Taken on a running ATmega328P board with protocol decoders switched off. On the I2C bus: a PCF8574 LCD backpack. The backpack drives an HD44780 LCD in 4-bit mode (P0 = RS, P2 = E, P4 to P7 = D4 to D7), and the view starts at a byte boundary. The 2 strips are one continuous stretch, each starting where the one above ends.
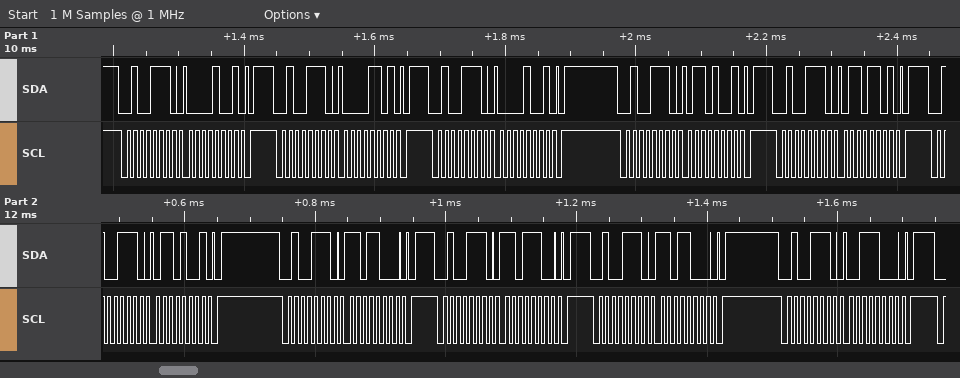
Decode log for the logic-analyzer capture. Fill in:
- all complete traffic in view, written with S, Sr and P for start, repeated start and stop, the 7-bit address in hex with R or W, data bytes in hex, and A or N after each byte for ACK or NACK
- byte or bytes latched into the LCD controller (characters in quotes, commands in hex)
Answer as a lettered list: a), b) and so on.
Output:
a) S 27W A 09 A P S 27W A 0D A P S 27W A 09 A P S 27W A 69 A P S 27W A 6D A P S 27W A 69 A P S 27W A D8 A P S 27W A DC A P S 27W A D8 A P S 27W A 38 A P
b) data 0x06
